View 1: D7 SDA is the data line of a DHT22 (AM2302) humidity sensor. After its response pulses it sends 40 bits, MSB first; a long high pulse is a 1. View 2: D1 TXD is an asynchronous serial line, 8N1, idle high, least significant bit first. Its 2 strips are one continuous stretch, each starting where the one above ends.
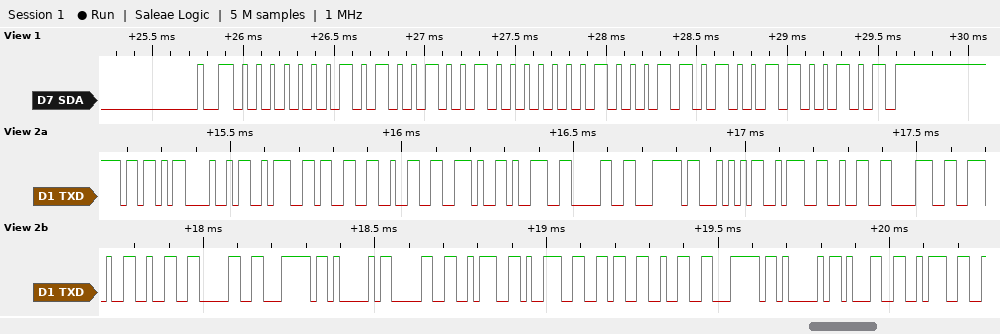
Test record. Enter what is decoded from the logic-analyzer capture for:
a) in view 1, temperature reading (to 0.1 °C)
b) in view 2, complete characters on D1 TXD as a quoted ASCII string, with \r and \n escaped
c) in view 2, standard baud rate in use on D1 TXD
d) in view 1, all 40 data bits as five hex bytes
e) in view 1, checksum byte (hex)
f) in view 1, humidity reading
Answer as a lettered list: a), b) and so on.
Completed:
a) 28.2 °C
b) "[H:32.90|T:28.20|A0:962|A1:"
c) 57600 baud
d) 01 49 01 1A 65
e) 0x65
f) 32.9 %
